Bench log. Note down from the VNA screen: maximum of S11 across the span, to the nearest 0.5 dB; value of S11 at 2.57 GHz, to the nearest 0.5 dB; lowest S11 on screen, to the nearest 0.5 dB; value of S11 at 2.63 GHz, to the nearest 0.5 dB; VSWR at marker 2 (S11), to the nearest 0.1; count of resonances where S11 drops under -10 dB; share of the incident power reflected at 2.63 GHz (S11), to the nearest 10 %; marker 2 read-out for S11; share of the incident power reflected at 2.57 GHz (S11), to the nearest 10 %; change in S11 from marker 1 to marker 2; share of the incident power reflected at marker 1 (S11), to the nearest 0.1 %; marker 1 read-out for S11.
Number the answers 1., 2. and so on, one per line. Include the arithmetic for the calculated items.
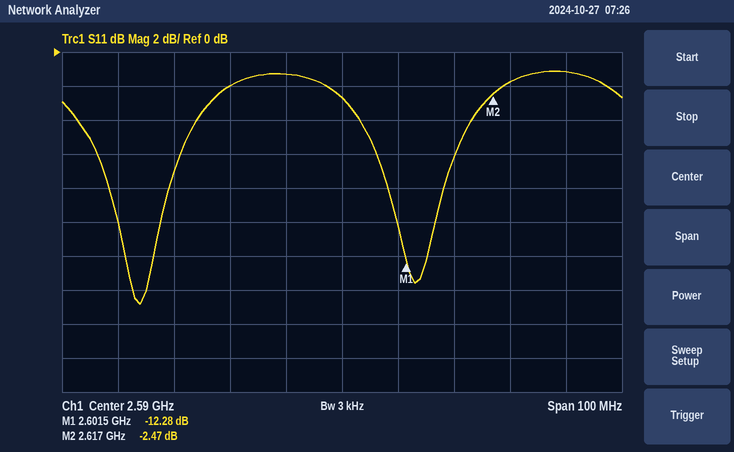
1. -1.0 dB
2. -2.0 dB
3. -15.0 dB
4. -1.0 dB
5. (1 + 0.7525)/(1 − 0.7525) ≈ 7.1
6. 2
7. 10^(-1/10) ≈ 79.4 %, so 80 % to the nearest 10 %
8. -2.47 dB
9. 10^(-2/10) ≈ 63.1 %, so 60 % to the nearest 10 %
10. -2.47 − (-12.28) = 9.81 dB
11. 10^(-12.28/10) ≈ 5.9 %
12. -12.28 dB
